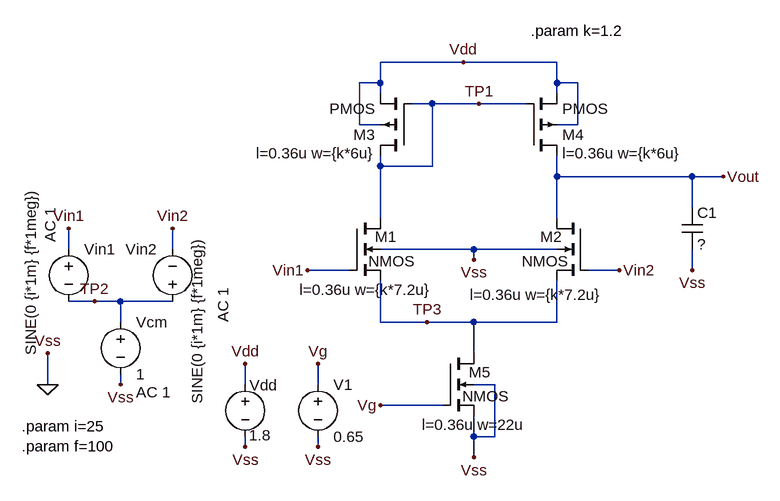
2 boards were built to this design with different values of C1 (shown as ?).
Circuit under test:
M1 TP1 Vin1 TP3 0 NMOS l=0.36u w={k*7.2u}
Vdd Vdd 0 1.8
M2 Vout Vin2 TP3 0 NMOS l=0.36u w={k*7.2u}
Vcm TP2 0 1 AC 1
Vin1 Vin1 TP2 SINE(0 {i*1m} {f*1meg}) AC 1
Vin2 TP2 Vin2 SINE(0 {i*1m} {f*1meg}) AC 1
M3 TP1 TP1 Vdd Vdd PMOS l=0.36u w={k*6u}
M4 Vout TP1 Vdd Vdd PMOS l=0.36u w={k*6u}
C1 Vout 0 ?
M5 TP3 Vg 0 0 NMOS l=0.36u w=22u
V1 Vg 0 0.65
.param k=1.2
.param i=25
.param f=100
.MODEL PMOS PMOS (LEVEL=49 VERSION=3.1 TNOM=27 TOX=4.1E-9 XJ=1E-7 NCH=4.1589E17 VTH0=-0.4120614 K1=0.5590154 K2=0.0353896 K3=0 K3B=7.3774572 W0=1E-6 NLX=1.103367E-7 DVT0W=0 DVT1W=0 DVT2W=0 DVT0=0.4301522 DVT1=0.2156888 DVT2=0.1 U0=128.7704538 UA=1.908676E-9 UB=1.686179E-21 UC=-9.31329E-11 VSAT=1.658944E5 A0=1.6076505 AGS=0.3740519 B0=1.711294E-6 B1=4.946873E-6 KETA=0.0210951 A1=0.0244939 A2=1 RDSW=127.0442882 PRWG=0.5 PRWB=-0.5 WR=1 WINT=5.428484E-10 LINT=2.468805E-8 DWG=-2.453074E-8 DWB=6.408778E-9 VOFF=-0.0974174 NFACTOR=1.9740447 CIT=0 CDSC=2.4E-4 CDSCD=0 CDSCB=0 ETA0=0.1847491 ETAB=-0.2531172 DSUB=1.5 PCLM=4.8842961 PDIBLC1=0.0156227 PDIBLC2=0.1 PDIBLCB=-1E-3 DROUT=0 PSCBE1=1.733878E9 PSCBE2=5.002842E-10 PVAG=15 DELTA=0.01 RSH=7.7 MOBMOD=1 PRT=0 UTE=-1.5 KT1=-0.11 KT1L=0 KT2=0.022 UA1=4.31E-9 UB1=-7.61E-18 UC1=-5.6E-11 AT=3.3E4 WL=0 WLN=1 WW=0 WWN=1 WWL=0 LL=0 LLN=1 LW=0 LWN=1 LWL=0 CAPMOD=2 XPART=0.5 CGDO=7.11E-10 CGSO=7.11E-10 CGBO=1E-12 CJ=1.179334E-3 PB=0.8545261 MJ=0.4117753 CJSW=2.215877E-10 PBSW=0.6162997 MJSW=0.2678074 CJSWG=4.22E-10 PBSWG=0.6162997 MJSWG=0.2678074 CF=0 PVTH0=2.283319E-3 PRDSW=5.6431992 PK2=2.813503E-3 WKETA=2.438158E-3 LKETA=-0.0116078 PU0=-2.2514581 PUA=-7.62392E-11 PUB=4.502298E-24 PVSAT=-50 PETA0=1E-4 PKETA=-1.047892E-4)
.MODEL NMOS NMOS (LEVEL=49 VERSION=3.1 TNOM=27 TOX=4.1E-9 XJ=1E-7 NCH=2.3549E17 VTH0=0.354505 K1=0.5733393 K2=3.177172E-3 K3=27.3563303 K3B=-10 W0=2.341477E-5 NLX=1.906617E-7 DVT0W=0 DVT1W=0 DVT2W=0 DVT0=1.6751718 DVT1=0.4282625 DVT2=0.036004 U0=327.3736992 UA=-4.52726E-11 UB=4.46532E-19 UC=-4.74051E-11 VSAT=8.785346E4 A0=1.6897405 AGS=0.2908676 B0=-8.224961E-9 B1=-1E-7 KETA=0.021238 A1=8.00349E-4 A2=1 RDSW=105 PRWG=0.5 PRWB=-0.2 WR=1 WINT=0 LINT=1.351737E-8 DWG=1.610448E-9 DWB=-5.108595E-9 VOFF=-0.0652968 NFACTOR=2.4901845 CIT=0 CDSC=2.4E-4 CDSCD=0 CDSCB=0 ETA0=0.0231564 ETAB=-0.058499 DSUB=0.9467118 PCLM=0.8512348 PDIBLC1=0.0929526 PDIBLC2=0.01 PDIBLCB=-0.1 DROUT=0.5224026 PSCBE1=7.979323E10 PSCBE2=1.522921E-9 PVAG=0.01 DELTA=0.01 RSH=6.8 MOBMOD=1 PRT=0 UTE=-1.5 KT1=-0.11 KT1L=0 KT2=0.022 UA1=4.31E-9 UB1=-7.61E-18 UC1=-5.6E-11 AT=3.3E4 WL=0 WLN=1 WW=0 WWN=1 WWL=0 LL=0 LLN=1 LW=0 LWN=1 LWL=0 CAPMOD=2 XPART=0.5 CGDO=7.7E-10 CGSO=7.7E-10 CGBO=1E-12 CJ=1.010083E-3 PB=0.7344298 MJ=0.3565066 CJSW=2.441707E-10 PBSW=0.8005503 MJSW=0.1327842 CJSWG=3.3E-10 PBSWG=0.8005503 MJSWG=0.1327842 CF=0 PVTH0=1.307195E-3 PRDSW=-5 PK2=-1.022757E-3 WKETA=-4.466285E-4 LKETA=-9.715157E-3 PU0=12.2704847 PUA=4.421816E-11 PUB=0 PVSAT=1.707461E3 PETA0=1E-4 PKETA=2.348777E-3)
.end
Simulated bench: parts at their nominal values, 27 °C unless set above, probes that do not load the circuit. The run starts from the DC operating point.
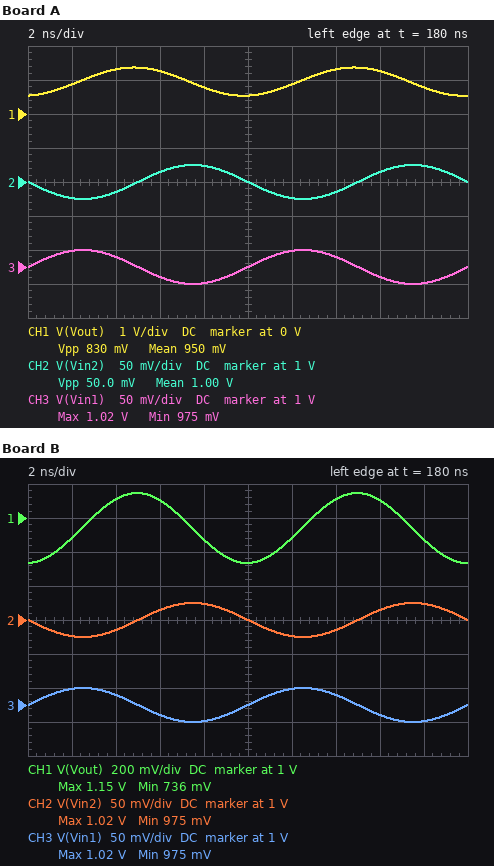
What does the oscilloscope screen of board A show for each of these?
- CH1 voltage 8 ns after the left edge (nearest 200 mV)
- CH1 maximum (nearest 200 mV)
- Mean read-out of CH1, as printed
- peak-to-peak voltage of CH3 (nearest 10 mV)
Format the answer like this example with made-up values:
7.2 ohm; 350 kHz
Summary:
800 mV; 1.4 V; 950 mV; 50 mV
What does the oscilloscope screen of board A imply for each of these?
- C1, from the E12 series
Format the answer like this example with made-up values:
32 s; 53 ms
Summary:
180 fF
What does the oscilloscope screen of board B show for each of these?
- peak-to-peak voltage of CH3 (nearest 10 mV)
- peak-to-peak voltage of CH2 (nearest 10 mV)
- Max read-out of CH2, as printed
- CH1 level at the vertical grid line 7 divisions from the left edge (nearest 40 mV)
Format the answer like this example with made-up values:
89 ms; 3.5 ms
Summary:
50 mV; 50 mV; 1.02 V; 1.12 V
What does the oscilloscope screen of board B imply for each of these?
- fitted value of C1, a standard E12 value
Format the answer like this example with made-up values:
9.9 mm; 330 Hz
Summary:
390 fF
